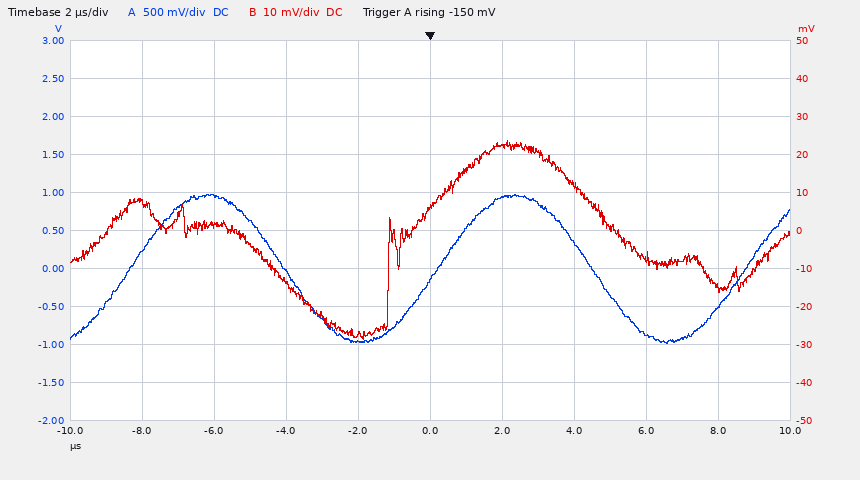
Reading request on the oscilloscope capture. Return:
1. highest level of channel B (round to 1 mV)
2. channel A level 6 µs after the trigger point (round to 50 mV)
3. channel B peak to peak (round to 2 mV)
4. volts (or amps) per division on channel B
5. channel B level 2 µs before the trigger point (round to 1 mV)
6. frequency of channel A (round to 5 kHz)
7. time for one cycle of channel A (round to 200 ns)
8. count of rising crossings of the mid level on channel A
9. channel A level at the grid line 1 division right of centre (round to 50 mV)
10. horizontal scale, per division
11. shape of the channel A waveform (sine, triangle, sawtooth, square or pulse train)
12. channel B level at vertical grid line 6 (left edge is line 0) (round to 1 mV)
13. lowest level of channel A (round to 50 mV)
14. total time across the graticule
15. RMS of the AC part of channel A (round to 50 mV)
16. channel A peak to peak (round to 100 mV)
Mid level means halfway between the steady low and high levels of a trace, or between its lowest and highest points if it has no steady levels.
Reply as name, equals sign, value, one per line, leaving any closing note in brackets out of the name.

highest level of channel B = 24 mV
channel A level 6 µs after the trigger point = -850 mV
channel B peak to peak = 52 mV
volts (or amps) per division on channel B = 10 mV
channel B level 2 µs before the trigger point = -27 mV
frequency of channel A = 115 kHz
time for one cycle of channel A = 8.6 µs
count of rising crossings of the mid level on channel A = 3
channel A level at the grid line 1 division right of centre = 950 mV
horizontal scale, per division = 2 µs
shape of the channel A waveform = sine
channel B level at vertical grid line 6 (left edge is line 0) = 22 mV
lowest level of channel A = -1.00 V
total time across the graticule = 20 µs
RMS of the AC part of channel A = 700 mV
channel A peak to peak = 2.00 V
